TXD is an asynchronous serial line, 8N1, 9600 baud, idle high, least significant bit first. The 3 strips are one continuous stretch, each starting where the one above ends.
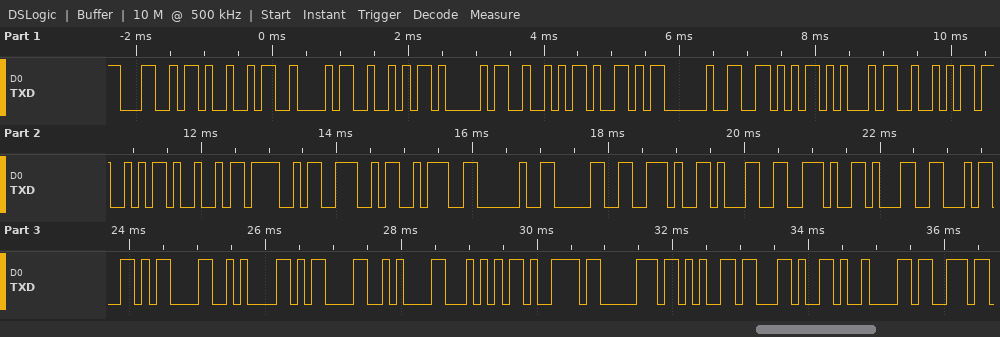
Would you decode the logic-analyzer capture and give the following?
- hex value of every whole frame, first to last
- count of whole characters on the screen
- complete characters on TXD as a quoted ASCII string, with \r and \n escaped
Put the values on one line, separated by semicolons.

4C 49 42 52 41 52 59 20 56 45 52 53 49 4F 4E 3A 20 30 2E 31 2E 31 34 0D 0A 0D 0A 54 79 70 65 2C 09 73; 34; "LIBRARY VERSION: 0.1.14\r\n\r\nType,\ts"
